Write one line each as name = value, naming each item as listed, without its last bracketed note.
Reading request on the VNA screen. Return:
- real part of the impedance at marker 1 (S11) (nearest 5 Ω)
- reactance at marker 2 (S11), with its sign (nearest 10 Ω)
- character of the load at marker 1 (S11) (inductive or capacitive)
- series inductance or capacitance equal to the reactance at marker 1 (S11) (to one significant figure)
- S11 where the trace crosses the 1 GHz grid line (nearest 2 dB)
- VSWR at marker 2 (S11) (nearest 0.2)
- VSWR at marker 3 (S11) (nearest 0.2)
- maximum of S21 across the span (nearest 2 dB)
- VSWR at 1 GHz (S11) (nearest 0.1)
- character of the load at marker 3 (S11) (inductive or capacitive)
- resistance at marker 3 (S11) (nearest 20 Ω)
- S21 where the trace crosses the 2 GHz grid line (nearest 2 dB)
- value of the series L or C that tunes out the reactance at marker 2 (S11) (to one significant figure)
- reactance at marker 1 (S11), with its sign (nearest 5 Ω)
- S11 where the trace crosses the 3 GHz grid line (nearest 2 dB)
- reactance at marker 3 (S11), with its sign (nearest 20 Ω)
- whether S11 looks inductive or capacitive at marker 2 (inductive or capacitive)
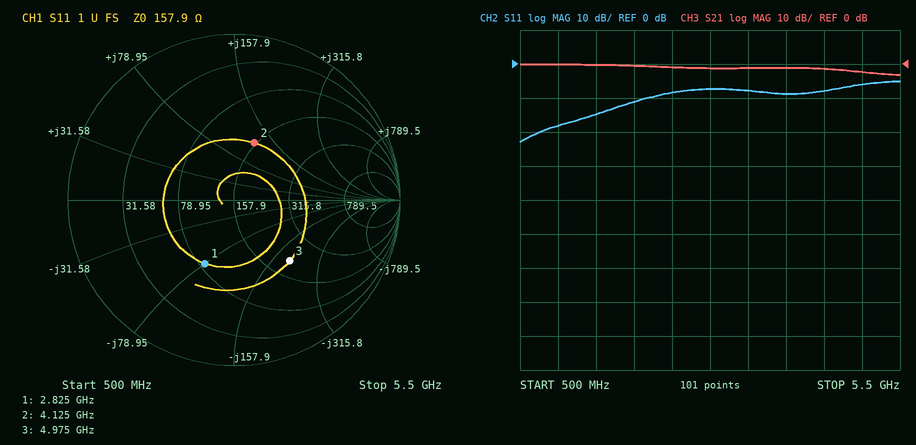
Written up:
real part of the impedance at marker 1 (S11) = 85 Ω
reactance at marker 2 (S11), with its sign = +120 Ω
character of the load at marker 1 (S11) = capacitive
series inductance or capacitance equal to the reactance at marker 1 (S11) = 700 fF
S11 where the trace crosses the 1 GHz grid line = -18 dB
VSWR at marker 2 (S11) = 2.2
VSWR at marker 3 (S11) = 3.0
maximum of S21 across the span = 0 dB
VSWR at 1 GHz (S11) = 1.3
character of the load at marker 3 (S11) = capacitive
resistance at marker 3 (S11) = 200 Ω
S21 where the trace crosses the 2 GHz grid line = 0 dB
value of the series L or C that tunes out the reactance at marker 2 (S11) = 300 fF
reactance at marker 1 (S11), with its sign = -80 Ω
S11 where the trace crosses the 3 GHz grid line = -8 dB
reactance at marker 3 (S11), with its sign = -200 Ω
whether S11 looks inductive or capacitive at marker 2 = inductive
